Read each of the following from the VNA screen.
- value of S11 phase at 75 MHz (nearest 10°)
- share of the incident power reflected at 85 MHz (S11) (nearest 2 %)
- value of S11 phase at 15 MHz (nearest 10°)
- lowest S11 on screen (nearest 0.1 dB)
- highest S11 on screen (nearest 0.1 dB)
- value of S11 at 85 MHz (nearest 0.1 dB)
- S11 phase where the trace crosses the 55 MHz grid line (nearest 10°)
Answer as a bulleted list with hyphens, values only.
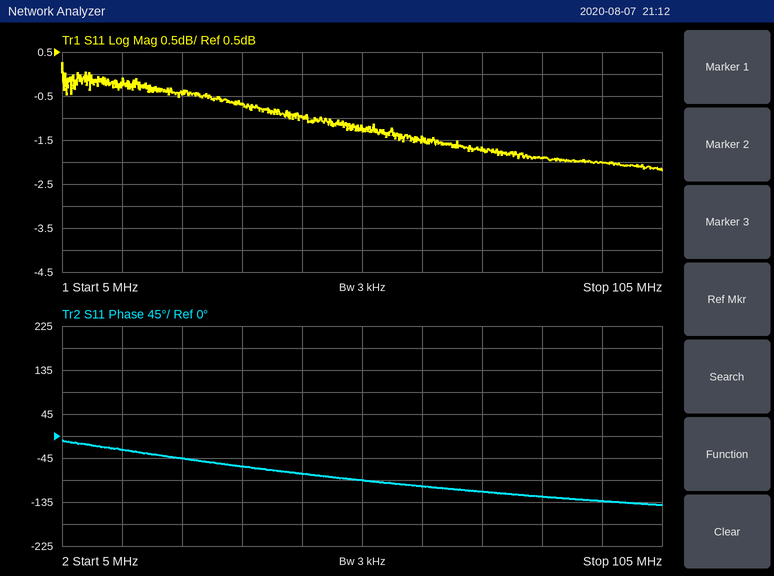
- -110°
- 64 %
- -30°
- -2.2 dB
- 0.3 dB
- -1.9 dB
- -90°
